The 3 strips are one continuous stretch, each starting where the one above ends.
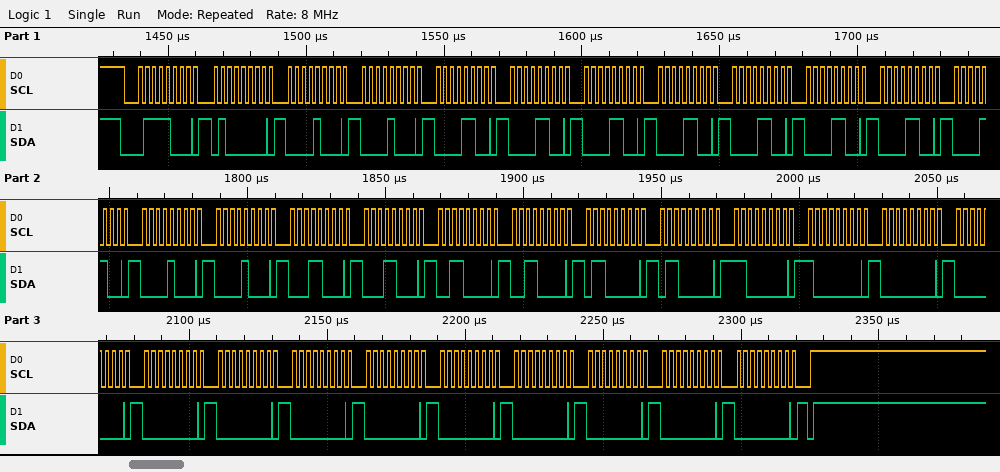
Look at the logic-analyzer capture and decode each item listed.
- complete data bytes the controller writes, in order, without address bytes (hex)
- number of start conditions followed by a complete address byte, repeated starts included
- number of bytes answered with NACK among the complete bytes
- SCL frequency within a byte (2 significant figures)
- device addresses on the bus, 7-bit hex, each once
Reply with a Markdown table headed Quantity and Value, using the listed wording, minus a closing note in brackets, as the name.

| Quantity | Value |
|---|---|
| complete data bytes the controller writes, in order, without address bytes | 40 08 08 0C 0C 0C 0C 0C 0C 0C 0C 08 08 18 18 30 30 60 60 C0 80 00 00 00 00 00 00 00 00 00 00 00 |
| number of start conditions followed by a complete address byte, repeated starts included | 1 |
| number of bytes answered with NACK among the complete bytes | 0 |
| SCL frequency within a byte | 400 kHz |
| device addresses on the bus, 7-bit hex, each once | 0x3C |
